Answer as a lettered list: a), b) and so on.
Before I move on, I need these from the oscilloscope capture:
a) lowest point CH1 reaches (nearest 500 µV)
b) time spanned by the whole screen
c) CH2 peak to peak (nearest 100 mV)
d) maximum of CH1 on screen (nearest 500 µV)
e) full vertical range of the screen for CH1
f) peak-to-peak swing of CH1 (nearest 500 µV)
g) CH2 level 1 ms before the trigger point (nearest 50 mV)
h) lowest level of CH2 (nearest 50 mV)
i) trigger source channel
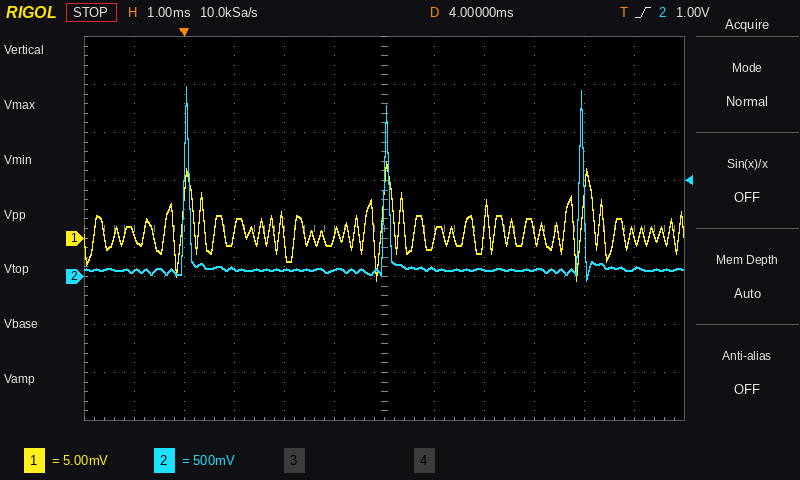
a) -4.5 mV
b) 12 ms
c) 2.00 V
d) 8.0 mV
e) 40 mV
f) 12.5 mV
g) 50 mV
h) -50 mV
i) CH2
